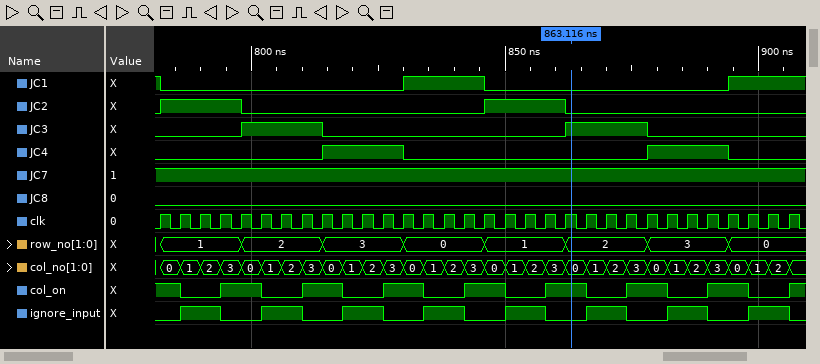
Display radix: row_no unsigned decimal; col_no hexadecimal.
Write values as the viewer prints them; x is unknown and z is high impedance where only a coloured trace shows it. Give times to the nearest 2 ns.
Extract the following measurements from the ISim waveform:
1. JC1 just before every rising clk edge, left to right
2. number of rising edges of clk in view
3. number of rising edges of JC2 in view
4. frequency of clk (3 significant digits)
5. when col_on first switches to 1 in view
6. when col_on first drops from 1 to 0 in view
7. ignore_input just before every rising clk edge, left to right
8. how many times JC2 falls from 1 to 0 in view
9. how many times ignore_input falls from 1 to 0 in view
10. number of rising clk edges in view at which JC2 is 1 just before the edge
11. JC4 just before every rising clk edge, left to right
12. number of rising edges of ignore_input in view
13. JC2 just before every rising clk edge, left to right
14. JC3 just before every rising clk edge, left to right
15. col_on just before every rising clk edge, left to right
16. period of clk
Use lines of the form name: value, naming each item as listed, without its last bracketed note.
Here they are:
JC1 just before every rising clk edge, left to right: 1 0 0 0 0 0 0 0 0 0 0 0 0 1 1 1 1 0 0 0 0 0 0 0 0 0 0 0 0 1 1 1
number of rising edges of clk in view: 32
number of rising edges of JC2 in view: 2
frequency of clk: 250 MHz
when col_on first switches to 1 in view: 794 ns
when col_on first drops from 1 to 0 in view: 786 ns
ignore_input just before every rising clk edge, left to right: 0 0 1 1 0 0 1 1 0 0 1 1 0 0 1 1 0 0 1 1 0 0 1 1 0 0 1 1 0 0 1 1
how many times JC2 falls from 1 to 0 in view: 2
how many times ignore_input falls from 1 to 0 in view: 8
number of rising clk edges in view at which JC2 is 1 just before the edge: 8
JC4 just before every rising clk edge, left to right: 0 0 0 0 0 0 0 0 0 1 1 1 1 0 0 0 0 0 0 0 0 0 0 0 0 1 1 1 1 0 0 0
number of rising edges of ignore_input in view: 8
JC2 just before every rising clk edge, left to right: 0 1 1 1 1 0 0 0 0 0 0 0 0 0 0 0 0 1 1 1 1 0 0 0 0 0 0 0 0 0 0 0
JC3 just before every rising clk edge, left to right: 0 0 0 0 0 1 1 1 1 0 0 0 0 0 0 0 0 0 0 0 0 1 1 1 1 0 0 0 0 0 0 0
col_on just before every rising clk edge, left to right: 1 1 0 0 1 1 0 0 1 1 0 0 1 1 0 0 1 1 0 0 1 1 0 0 1 1 0 0 1 1 0 0
period of clk: 4 ns
